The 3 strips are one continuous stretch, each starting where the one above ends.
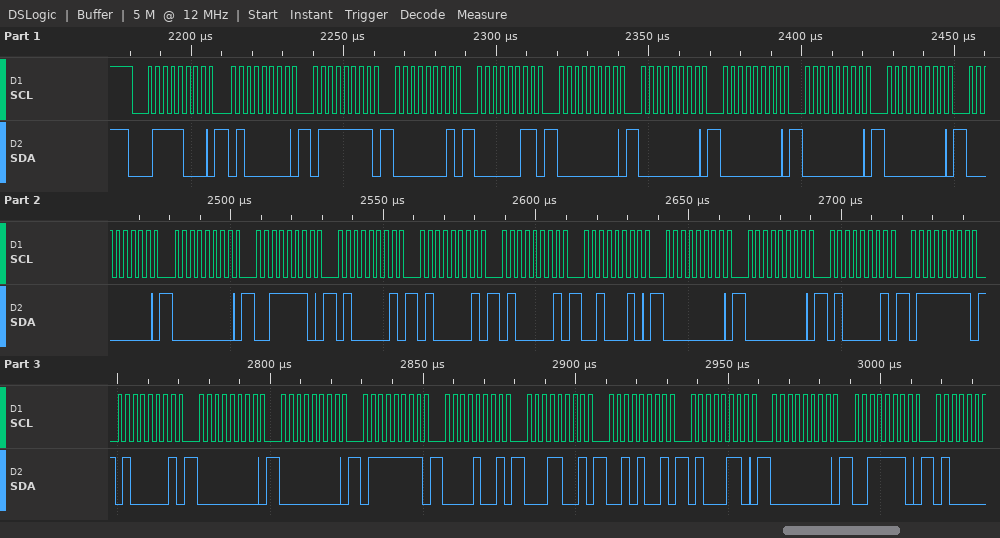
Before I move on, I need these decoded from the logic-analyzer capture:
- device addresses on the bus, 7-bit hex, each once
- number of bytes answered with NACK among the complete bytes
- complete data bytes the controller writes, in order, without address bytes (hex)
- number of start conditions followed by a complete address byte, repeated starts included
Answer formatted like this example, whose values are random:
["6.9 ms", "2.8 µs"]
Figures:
["0x3C", "0", "40 7F 01 03 00 00 00 00 00 00 00 3E 41 41 41 22 00 00 41 7F 41 00 00 7F 09 19 29 46 00 3E", "1"]
